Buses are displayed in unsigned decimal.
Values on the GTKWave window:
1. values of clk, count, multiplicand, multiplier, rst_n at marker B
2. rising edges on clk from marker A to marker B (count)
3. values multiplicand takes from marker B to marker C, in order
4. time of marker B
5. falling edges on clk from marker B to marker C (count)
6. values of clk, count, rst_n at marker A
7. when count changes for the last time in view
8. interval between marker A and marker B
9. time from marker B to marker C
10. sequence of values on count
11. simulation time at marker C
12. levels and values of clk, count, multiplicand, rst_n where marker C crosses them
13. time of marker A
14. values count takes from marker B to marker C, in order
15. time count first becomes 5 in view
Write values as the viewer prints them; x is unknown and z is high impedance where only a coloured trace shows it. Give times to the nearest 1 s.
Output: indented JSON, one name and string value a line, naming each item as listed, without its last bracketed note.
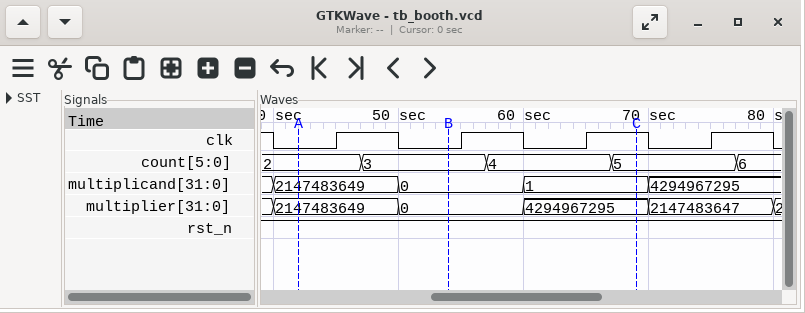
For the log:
{
  "values of clk, count, multiplicand, multiplier, rst_n at marker B": "clk=0, count=3, multiplicand=0, multiplier=0, rst_n=1",
  "rising edges on clk from marker A to marker B": "1",
  "values multiplicand takes from marker B to marker C, in order": "0, 1",
  "time of marker B": "54 s",
  "falling edges on clk from marker B to marker C": "1",
  "values of clk, count, rst_n at marker A": "clk=0, count=2, rst_n=1",
  "when count changes for the last time in view": "77 s",
  "interval between marker A and marker B": "12 s",
  "time from marker B to marker C": "15 s",
  "sequence of values on count": "2, 3, 4, 5, 6",
  "simulation time at marker C": "69 s",
  "levels and values of clk, count, multiplicand, rst_n where marker C crosses them": "clk=1, count=5, multiplicand=1, rst_n=1",
  "time of marker A": "42 s",
  "values count takes from marker B to marker C, in order": "3, 4, 5",
  "time count first becomes 5 in view": "67 s"
}
